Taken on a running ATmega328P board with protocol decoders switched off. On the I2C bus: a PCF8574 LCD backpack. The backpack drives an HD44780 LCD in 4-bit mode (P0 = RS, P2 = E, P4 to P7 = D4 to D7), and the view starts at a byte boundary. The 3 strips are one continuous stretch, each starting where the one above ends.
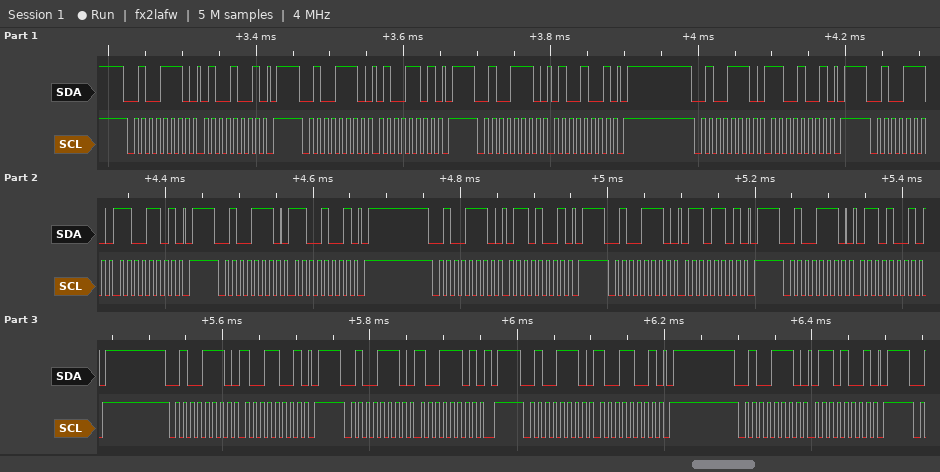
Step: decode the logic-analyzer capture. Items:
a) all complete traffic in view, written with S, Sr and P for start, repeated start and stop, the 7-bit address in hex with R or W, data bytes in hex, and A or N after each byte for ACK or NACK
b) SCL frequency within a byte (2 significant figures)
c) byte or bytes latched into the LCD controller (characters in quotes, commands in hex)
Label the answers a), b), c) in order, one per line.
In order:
a) S 27W A 49 A P S 27W A 4D A P S 27W A 49 A P S 27W A C9 A P S 27W A CD A P S 27W A C9 A P S 27W A 69 A P S 27W A 6D A P S 27W A 69 A P S 27W A 99 A P S 27W A 9D A P S 27W A 99 A P S 27W A 69 A P
b) 100 kHz
c) 'L' 'i'
